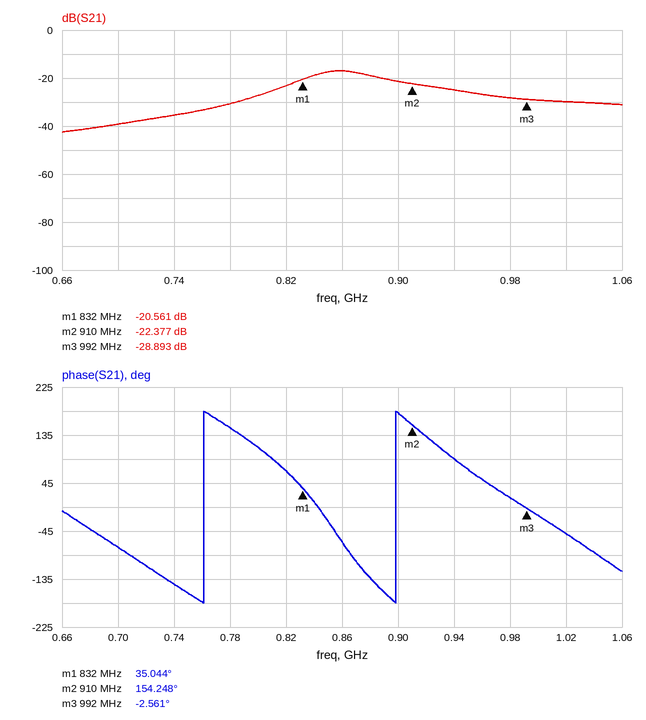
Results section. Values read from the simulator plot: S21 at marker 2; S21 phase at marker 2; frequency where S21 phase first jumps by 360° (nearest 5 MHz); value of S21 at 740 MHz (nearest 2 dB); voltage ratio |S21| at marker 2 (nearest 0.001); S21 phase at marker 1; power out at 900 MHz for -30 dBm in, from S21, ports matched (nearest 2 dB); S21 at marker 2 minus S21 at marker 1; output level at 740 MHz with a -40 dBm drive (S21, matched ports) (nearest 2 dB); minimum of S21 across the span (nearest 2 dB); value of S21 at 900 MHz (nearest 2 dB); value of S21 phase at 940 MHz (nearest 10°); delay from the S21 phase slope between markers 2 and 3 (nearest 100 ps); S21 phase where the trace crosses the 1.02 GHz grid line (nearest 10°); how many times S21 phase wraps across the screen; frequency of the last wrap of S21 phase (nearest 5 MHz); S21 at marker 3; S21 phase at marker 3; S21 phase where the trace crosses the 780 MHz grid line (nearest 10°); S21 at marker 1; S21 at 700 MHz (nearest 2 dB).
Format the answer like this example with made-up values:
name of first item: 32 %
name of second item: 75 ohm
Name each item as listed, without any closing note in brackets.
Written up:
S21 at marker 2: -22.377 dB
S21 phase at marker 2: 154.248°
frequency where S21 phase first jumps by 360°: 760 MHz
value of S21 at 740 MHz: -36 dB
voltage ratio |S21| at marker 2: 0.076
S21 phase at marker 1: 35.044°
power out at 900 MHz for -30 dBm in, from S21, ports matched: -52 dBm
S21 at marker 2 minus S21 at marker 1: -1.816 dB
output level at 740 MHz with a -40 dBm drive (S21, matched ports): -76 dBm
minimum of S21 across the span: -42 dB
value of S21 at 900 MHz: -22 dB
value of S21 phase at 940 MHz: 90°
delay from the S21 phase slope between markers 2 and 3: 5.3 ns
S21 phase where the trace crosses the 1.02 GHz grid line: -50°
how many times S21 phase wraps across the screen: 2
frequency of the last wrap of S21 phase: 900 MHz
S21 at marker 3: -28.893 dB
S21 phase at marker 3: -2.561°
S21 phase where the trace crosses the 780 MHz grid line: 150°
S21 at marker 1: -20.561 dB
S21 at 700 MHz: -40 dB
